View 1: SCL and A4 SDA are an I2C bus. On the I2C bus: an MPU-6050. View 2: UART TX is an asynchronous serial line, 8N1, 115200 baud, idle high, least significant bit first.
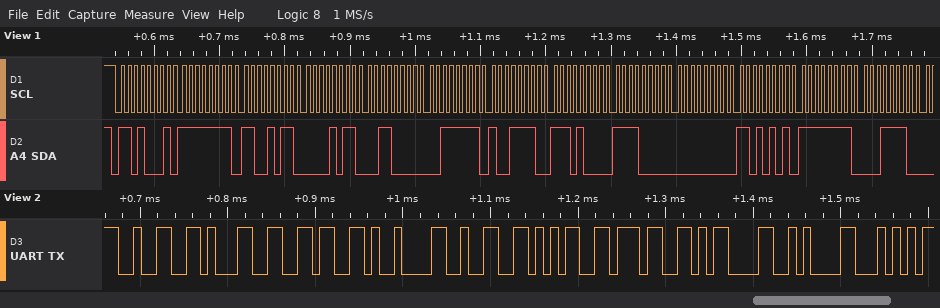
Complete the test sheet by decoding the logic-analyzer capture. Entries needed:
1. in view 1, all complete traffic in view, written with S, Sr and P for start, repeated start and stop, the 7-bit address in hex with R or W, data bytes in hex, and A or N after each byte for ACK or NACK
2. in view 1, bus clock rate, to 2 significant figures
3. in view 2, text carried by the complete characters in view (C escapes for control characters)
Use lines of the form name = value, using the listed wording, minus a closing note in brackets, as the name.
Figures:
in view 1, all complete traffic in view, written with S, Sr and P for start, repeated start and stop, the 7-bit address in hex with R or W, data bytes in hex, and A or N after each byte for ACK or NACK = S 68R A FF A CB A 0B A 30 A 3F A 9E A E8 A F0 A 00 A D5 A FF A 1E A
in view 1, bus clock rate, to 2 significant figures = 100 kHz
in view 2, text carried by the complete characters in view = "216\t257\r\nT"
